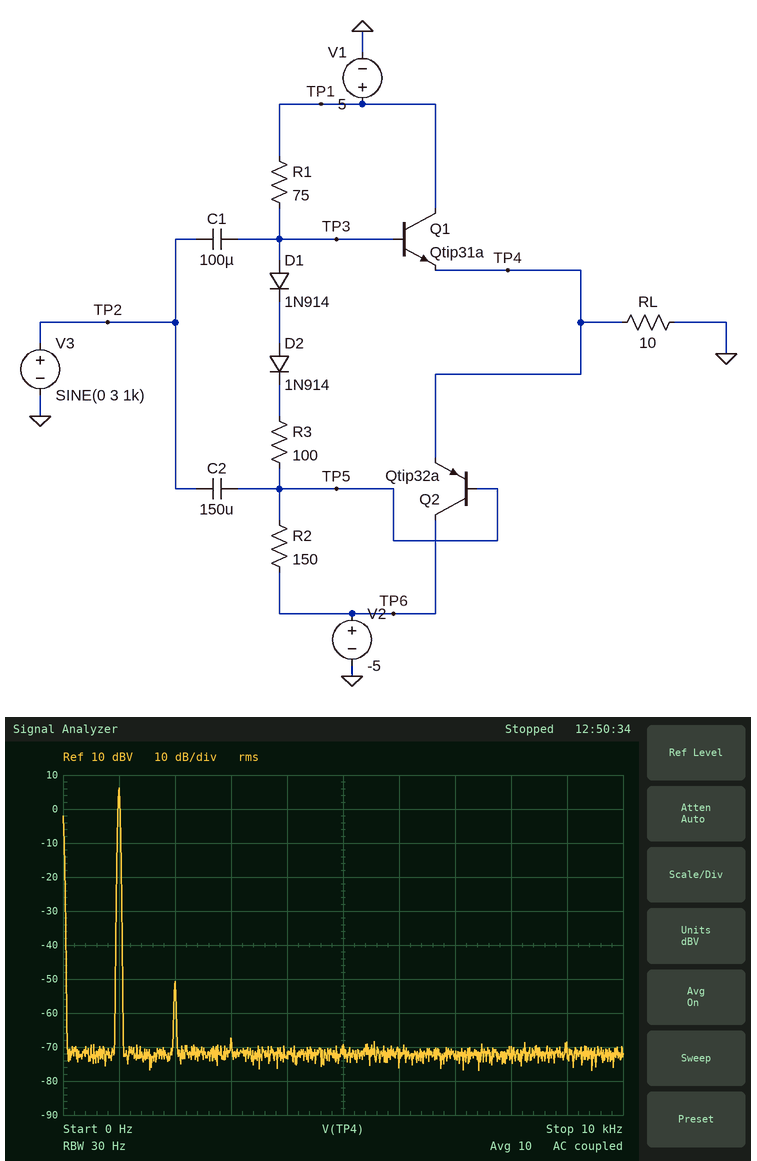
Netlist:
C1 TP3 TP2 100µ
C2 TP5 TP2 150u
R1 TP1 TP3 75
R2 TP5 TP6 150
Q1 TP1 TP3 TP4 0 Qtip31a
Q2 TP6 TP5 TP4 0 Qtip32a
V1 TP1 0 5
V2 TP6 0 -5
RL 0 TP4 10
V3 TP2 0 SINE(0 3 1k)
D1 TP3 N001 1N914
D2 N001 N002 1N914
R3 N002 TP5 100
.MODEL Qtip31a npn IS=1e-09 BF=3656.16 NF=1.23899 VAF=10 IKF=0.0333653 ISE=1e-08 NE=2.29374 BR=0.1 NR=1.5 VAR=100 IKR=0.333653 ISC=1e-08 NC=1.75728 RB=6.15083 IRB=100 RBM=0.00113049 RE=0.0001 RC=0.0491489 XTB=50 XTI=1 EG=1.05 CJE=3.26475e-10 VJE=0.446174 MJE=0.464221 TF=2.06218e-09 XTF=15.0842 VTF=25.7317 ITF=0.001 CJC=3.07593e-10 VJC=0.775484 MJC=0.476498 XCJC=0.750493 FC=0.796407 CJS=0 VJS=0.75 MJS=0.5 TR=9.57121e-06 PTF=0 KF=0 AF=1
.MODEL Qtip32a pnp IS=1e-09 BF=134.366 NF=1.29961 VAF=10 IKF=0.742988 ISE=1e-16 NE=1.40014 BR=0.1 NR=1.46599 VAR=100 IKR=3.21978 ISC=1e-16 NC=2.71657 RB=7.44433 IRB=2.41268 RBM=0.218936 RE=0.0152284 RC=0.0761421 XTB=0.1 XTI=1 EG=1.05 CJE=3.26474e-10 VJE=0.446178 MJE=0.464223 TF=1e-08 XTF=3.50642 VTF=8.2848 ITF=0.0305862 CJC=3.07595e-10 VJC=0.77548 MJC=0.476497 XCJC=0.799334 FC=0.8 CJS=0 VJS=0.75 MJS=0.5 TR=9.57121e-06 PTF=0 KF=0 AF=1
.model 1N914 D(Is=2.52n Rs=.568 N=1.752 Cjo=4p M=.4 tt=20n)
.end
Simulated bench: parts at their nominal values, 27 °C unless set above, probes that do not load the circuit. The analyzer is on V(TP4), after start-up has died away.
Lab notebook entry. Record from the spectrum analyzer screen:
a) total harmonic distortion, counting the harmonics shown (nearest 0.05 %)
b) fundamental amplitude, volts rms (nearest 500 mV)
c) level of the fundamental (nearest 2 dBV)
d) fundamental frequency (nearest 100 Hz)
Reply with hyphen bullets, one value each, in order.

- 0.15 %
- 2.0 V
- 6 dBV
- 1.0 kHz
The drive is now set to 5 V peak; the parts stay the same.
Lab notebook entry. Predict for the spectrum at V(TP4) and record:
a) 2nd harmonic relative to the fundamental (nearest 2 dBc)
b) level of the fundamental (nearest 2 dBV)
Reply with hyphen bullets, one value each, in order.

- -32 dBc
- 10 dBV
